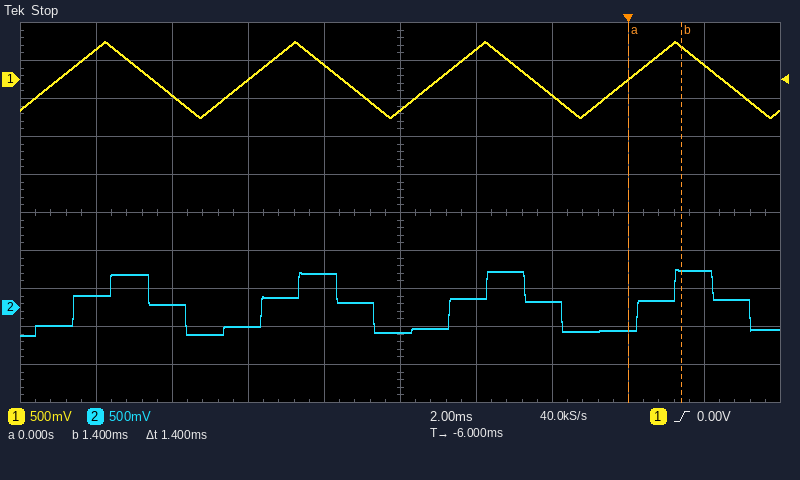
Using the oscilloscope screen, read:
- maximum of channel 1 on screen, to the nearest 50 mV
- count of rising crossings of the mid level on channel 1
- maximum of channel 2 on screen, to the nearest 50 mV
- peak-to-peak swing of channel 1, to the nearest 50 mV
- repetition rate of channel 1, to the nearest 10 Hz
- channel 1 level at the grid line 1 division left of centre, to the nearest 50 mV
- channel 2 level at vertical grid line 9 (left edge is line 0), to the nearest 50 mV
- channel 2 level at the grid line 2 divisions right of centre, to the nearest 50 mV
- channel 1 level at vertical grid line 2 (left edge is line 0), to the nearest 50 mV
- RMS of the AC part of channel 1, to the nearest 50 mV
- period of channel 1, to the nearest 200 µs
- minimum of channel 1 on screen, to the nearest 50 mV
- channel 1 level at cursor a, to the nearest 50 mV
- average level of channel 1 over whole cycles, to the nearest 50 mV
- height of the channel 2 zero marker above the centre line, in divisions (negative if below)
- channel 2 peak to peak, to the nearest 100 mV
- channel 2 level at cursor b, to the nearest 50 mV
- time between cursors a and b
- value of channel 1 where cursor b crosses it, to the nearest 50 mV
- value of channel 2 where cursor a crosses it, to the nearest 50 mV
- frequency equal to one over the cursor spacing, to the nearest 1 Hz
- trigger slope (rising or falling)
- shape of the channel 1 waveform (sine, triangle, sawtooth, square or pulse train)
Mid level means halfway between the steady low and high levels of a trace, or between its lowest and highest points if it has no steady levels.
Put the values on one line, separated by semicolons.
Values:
500 mV; 4; 500 mV; 1.00 V; 200 Hz; 200 mV; 500 mV; 100 mV; -200 mV; 300 mV; 5.0 ms; -500 mV; 0 mV; 0 mV; -2.5 div; 900 mV; 500 mV; 1.4 ms; 450 mV; -300 mV; 714 Hz; rising; triangle
